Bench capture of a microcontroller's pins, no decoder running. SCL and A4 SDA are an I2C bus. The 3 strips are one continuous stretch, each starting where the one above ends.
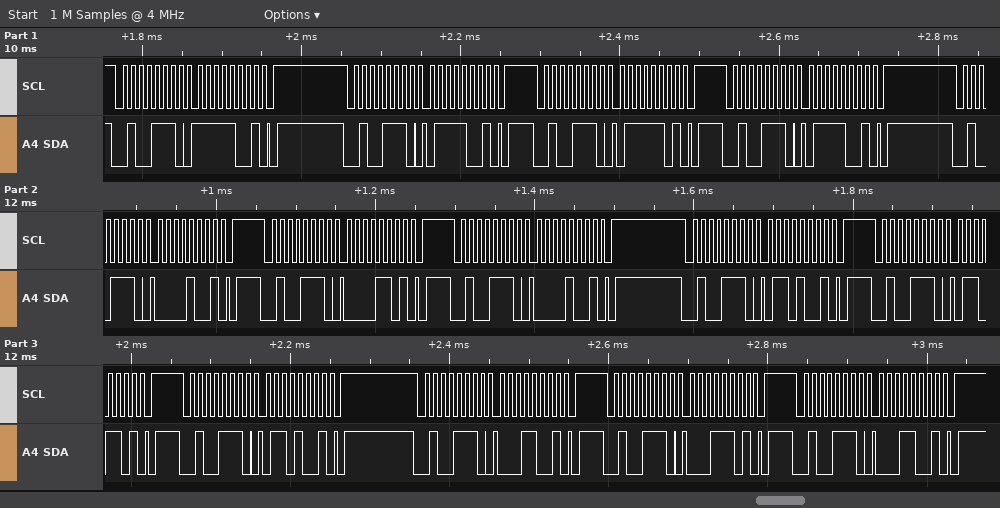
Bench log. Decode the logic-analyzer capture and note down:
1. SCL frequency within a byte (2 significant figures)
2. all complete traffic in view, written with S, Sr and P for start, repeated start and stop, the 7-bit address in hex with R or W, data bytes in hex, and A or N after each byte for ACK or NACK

100 kHz
S 27W A F9 A P S 27W A 79 A P S 27W A 7D A P S 27W A 79 A P S 27W A 09 A P S 27W A 0D A P S 27W A 09 A P S 27W A 69 A P S 27W A 6D A P S 27W A 69 A P S 27W A 19 A P S 27W A 1D A P S 27W A 19 A P
